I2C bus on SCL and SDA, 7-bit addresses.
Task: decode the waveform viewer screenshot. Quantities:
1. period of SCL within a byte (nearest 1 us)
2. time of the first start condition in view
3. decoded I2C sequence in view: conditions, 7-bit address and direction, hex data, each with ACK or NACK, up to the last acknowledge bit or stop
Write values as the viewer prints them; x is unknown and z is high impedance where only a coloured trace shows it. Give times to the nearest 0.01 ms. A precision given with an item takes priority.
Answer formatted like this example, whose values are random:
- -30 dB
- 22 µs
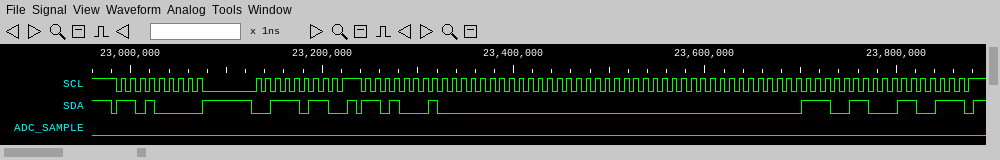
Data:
- 10 us
- 22.98 ms
- start, address 68 write ACK, 3B ACK, stop, start, address 68 read ACK, 00 ACK, 00 ACK, 00 ACK, 00 ACK, 73 ACK, 33 NACK, stop
